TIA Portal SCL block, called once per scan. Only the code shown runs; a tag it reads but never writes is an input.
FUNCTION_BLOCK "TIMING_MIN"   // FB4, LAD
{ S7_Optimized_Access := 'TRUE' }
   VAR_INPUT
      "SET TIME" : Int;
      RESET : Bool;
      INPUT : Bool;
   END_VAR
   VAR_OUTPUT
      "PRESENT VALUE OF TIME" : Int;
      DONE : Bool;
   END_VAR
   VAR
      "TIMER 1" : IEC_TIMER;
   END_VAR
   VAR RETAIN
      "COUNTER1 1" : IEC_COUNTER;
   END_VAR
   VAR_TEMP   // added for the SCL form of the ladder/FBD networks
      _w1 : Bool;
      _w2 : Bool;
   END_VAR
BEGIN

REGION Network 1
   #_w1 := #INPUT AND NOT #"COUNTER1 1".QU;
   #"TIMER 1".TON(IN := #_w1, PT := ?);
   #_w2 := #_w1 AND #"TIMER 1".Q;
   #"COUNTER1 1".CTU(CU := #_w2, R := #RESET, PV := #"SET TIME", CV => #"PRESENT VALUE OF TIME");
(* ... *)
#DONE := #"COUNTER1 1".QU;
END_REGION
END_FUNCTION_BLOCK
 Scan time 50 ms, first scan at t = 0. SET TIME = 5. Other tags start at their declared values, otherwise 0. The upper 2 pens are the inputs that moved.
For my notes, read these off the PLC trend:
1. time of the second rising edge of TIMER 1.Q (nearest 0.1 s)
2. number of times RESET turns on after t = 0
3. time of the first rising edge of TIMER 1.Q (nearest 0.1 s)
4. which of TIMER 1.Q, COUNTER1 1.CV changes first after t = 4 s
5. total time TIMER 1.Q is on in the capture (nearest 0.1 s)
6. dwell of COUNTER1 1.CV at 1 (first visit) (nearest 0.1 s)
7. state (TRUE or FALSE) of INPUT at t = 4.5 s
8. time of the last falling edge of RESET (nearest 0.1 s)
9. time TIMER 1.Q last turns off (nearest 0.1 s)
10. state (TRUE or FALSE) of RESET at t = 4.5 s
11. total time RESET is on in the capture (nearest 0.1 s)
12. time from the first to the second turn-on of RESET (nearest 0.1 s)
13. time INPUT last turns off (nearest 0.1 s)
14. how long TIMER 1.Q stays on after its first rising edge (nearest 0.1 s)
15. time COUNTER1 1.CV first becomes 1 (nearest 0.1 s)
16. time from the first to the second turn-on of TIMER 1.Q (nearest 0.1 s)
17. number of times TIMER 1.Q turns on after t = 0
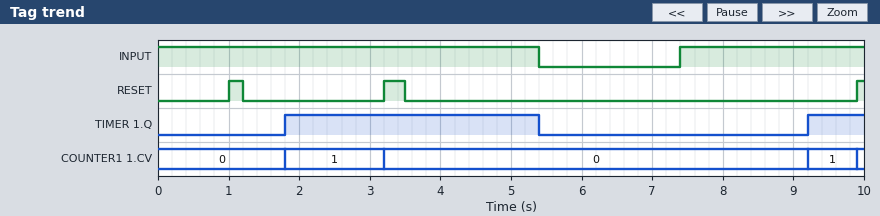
9.2 s
3
1.8 s
TIMER 1.Q
4.4 s
1.4 s
TRUE
3.5 s
5.4 s
FALSE
0.6 s
2.2 s
5.4 s
3.6 s
1.8 s
7.4 s
2
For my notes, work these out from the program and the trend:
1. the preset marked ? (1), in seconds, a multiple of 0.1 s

1.8 s
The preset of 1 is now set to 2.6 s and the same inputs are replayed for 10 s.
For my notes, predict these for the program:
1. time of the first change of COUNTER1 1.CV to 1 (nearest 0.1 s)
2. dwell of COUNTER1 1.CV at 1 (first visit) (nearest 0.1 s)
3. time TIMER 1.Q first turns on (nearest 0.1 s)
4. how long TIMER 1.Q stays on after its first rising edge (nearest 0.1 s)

2.6 s
0.6 s
2.6 s
2.8 s
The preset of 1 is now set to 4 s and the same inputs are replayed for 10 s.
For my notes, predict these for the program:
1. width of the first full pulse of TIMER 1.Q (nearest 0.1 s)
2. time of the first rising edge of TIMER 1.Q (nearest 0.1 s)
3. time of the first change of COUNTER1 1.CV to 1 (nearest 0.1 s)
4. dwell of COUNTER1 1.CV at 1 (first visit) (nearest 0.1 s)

1.4 s
4.0 s
4.0 s
5.9 s
